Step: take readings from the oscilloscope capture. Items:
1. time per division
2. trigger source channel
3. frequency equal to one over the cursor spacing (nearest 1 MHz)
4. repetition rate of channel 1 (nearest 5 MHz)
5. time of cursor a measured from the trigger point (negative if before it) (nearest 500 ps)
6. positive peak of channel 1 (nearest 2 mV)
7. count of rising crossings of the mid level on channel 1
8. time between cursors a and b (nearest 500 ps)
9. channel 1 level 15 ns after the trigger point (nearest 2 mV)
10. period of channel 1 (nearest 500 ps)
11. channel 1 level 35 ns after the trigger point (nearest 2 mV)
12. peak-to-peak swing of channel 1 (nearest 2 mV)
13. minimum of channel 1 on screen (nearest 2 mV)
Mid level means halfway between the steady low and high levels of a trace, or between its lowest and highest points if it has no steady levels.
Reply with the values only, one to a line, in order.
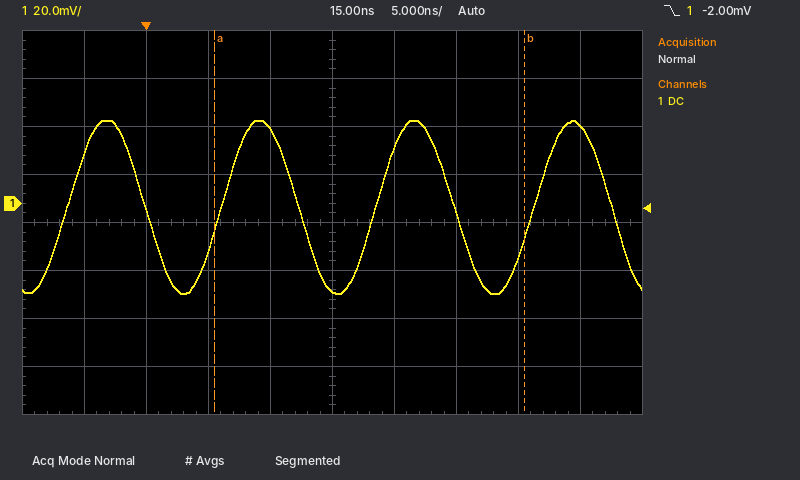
5 ns
channel 1
40 MHz
80 MHz
+5.5 ns
34 mV
4
25.0 ns
-36 mV
12.5 ns
32 mV
72 mV
-38 mV
